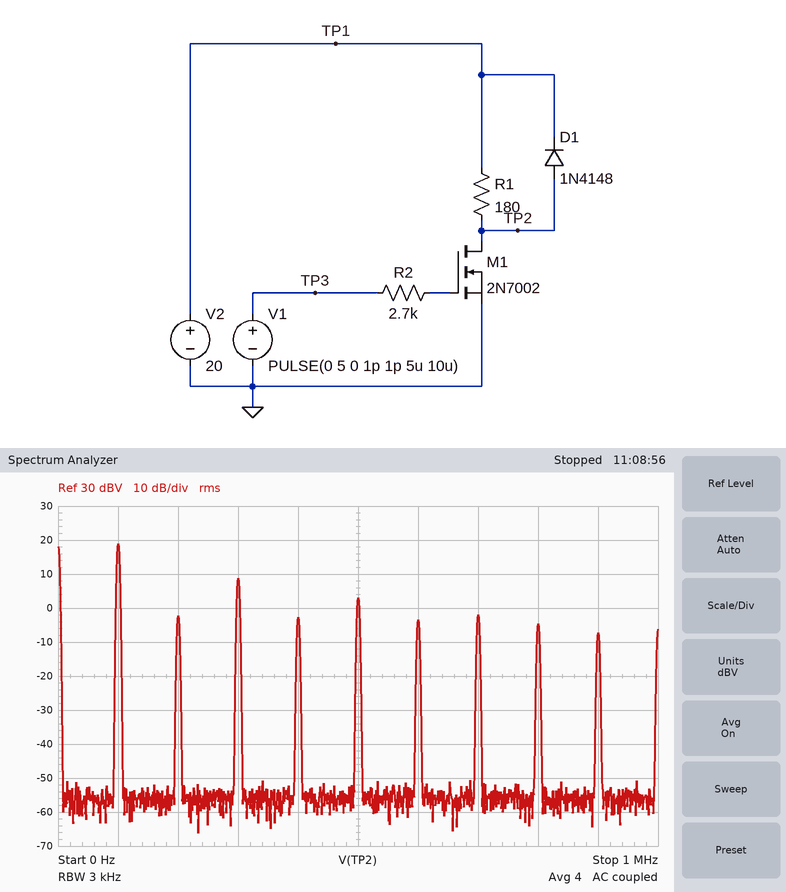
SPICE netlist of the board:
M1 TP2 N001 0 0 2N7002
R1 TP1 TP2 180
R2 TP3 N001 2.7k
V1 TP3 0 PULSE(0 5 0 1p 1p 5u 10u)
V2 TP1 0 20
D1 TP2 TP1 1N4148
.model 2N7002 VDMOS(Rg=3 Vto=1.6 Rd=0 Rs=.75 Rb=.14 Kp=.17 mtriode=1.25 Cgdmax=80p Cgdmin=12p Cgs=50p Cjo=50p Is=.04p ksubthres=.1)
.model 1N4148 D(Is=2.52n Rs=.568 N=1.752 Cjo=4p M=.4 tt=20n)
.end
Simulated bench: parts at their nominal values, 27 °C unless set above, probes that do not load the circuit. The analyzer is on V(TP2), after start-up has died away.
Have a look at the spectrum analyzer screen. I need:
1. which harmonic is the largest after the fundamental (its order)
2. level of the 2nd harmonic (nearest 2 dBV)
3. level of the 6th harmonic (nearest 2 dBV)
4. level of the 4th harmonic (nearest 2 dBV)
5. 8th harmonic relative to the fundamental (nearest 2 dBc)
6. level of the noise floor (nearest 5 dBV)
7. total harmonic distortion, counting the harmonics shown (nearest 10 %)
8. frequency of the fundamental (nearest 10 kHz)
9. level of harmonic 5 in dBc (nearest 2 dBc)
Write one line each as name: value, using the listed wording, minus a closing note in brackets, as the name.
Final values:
which harmonic is the largest after the fundamental: 3
level of the 2nd harmonic: -2 dBV
level of the 6th harmonic: -4 dBV
level of the 4th harmonic: -2 dBV
8th harmonic relative to the fundamental: -24 dBc
level of the noise floor: -55 dBV
total harmonic distortion, counting the harmonics shown: 40 %
frequency of the fundamental: 100 kHz
level of harmonic 5 in dBc: -16 dBc
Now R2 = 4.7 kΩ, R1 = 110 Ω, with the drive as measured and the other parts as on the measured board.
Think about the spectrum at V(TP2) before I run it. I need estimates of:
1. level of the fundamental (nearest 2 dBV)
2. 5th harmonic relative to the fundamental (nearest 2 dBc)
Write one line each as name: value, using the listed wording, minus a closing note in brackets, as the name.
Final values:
level of the fundamental: 18 dBV
5th harmonic relative to the fundamental: -18 dBc
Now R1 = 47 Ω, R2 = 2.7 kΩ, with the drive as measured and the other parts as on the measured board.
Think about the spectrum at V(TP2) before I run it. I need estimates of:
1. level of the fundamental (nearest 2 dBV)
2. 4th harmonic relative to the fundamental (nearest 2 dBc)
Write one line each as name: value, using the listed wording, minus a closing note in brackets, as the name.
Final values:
level of the fundamental: 18 dBV
4th harmonic relative to the fundamental: -32 dBc
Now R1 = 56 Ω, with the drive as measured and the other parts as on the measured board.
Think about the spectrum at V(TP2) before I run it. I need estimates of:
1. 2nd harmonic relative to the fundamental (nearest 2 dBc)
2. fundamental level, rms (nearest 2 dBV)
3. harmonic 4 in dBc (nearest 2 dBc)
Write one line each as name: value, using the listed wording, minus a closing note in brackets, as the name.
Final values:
2nd harmonic relative to the fundamental: -38 dBc
fundamental level, rms: 18 dBV
harmonic 4 in dBc: -34 dBc
